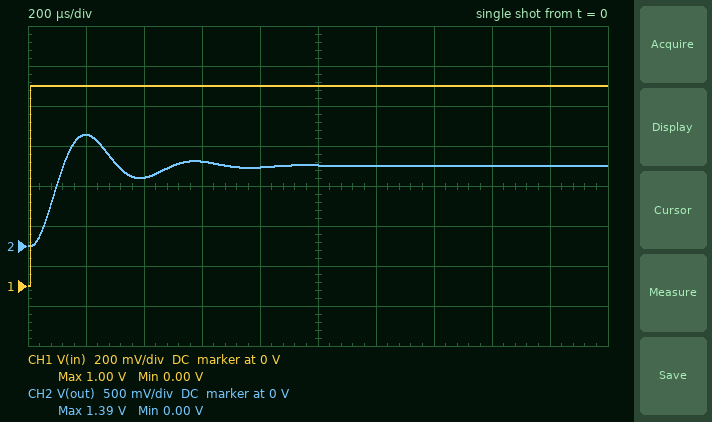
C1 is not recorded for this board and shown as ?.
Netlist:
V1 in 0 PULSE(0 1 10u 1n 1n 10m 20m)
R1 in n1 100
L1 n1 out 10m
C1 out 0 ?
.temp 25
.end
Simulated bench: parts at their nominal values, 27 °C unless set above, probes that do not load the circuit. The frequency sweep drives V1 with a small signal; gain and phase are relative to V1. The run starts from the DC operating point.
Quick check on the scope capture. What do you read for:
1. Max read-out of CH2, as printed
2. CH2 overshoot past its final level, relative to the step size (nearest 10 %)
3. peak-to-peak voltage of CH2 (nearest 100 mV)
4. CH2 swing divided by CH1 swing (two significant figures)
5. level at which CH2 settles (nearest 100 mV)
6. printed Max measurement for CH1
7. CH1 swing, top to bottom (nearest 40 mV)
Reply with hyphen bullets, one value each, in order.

- 1.39 V
- 40 %
- 1.4 V
- 1.4
- 1.0 V
- 1.00 V
- 1.00 V
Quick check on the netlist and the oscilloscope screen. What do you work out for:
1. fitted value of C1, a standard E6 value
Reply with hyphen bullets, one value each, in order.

- 330 nF
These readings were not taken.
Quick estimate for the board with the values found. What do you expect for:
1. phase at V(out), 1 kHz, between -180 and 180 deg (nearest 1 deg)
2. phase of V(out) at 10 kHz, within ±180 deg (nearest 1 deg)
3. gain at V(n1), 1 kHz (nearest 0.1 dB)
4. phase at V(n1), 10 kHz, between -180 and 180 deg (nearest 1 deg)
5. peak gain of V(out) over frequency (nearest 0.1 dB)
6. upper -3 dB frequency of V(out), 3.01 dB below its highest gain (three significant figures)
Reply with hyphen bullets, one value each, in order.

- -13 deg
- -170 deg
- -0.2 dB
- 10 deg
- 5.2 dB
- 3.26 kHz
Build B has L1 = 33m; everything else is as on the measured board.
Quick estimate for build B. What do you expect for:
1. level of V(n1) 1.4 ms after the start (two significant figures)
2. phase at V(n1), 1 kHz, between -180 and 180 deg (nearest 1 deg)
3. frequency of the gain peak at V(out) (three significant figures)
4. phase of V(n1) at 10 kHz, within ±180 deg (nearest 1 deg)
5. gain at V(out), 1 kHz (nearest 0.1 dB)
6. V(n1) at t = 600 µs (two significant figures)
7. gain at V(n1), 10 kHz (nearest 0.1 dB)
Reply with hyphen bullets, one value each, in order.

- 980 mV
- -20 deg
- 1.49 kHz
- 3 deg
- 4.3 dB
- 1.1 V
- 0 dB
